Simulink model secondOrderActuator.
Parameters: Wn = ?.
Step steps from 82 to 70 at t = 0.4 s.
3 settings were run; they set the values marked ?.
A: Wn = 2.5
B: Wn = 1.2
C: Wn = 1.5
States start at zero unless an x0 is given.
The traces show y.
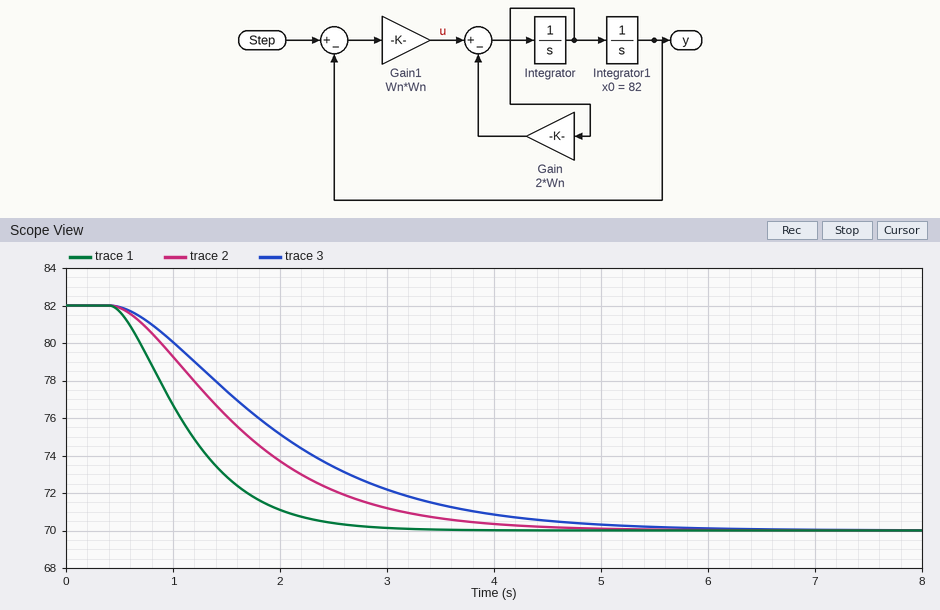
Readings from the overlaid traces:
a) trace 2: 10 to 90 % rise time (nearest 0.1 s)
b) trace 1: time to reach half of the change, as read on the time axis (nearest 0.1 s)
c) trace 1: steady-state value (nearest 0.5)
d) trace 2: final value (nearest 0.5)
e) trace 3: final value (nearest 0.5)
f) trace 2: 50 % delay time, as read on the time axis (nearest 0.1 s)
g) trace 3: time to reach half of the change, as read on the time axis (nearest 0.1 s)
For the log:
2.2 s
1.1 s
70.0
70.0
70.0
1.5 s
1.8 s
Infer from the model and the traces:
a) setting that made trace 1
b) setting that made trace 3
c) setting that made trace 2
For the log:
A
B
C
